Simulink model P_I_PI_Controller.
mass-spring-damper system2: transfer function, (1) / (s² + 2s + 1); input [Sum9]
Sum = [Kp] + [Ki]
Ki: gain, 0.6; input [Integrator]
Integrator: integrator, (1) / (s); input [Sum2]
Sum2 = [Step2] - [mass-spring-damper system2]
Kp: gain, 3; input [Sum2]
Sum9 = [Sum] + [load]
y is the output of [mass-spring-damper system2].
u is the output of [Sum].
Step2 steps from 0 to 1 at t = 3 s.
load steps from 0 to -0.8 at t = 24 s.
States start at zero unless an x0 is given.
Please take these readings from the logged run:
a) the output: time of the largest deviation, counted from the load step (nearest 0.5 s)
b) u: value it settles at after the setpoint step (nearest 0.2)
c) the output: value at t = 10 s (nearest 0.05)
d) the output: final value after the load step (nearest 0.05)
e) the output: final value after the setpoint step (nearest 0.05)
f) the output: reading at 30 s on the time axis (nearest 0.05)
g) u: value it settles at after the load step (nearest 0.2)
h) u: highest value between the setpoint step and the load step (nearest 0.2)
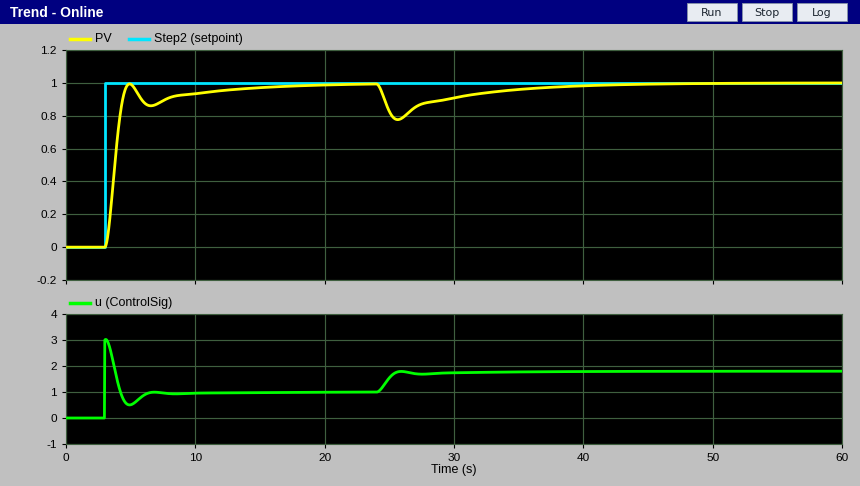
1.5 s
1.0
0.95
1.00
1.00
0.90
1.8
3.0
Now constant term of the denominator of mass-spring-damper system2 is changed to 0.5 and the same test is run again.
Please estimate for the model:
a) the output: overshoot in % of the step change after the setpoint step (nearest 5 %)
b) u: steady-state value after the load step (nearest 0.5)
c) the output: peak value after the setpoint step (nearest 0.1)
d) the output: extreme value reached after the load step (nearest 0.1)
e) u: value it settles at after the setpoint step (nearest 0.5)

10 %
1.5
1.1
0.8
0.5
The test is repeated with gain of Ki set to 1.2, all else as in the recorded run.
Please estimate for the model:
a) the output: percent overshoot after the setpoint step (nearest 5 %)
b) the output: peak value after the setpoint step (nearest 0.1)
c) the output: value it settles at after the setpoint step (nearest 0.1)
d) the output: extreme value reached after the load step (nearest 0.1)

10 %
1.1
1.0
0.8
